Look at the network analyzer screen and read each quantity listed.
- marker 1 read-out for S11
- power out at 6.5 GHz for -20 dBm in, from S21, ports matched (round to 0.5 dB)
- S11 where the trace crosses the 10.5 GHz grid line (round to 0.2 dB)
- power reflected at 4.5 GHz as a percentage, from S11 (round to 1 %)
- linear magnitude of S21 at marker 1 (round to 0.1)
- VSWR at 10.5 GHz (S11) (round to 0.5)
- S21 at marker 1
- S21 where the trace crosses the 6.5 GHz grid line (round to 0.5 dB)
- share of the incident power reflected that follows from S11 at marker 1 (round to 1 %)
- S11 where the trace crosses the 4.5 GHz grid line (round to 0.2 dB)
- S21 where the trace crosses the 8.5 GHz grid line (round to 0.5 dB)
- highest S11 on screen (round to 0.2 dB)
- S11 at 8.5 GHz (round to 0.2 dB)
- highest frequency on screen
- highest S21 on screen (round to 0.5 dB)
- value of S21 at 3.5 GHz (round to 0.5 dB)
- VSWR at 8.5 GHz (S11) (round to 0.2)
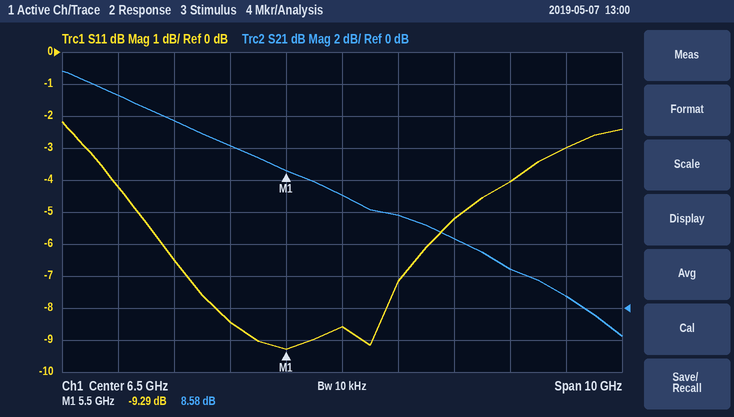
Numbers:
-9.29 dB
-13.0 dBm
-3.0 dB
14 %
2.7
6.0
8.58 dB
7.0 dB
12 %
-8.4 dB
4.5 dB
-2.2 dB
-5.2 dB
11.5 GHz
15.0 dB
11.5 dB
3.4
